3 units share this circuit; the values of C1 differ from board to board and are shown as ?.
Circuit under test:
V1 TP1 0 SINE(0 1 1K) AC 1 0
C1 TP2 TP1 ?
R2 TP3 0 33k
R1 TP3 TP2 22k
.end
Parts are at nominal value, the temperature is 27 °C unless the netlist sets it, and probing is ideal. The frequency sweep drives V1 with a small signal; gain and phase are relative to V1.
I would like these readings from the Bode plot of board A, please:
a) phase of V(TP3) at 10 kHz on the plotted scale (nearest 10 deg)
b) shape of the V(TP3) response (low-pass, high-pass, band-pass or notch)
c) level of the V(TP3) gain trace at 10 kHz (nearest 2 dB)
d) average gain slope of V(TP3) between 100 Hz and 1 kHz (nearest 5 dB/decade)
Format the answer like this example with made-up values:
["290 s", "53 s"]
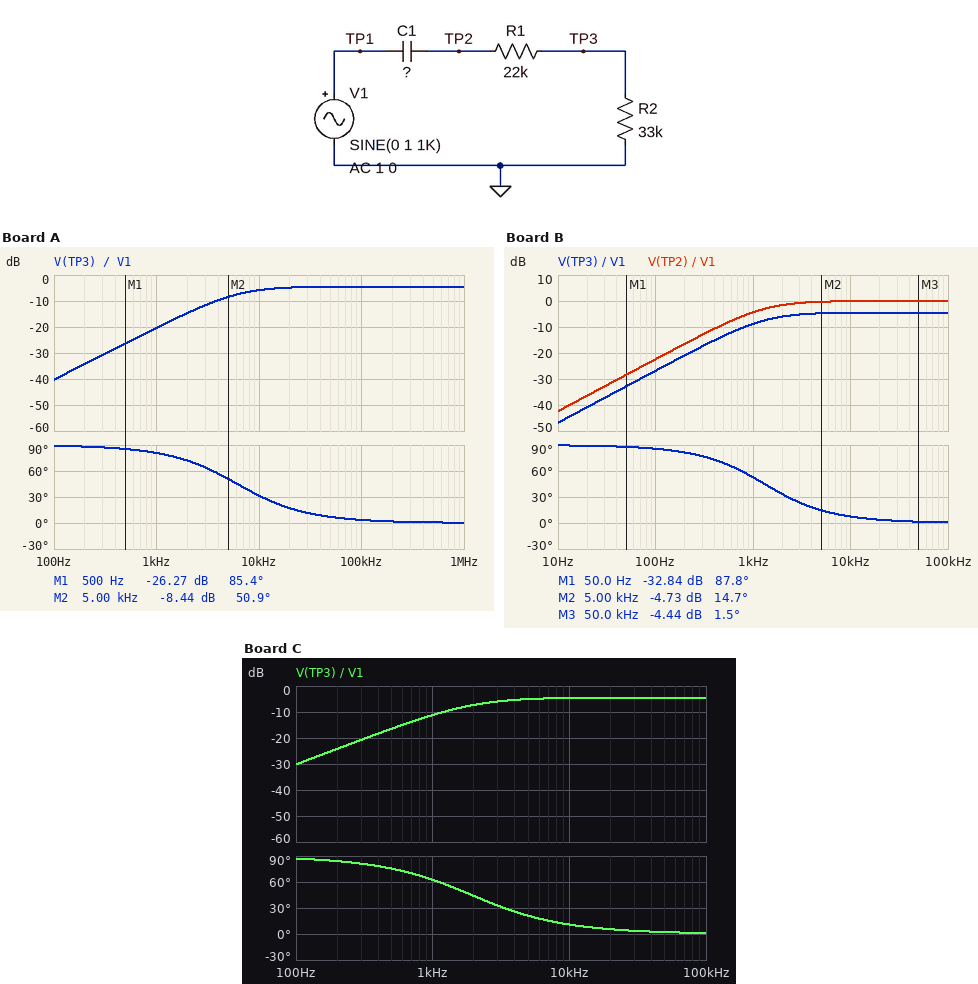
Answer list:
["30 deg", "high-pass", "-6 dB", "20 dB/decade"]
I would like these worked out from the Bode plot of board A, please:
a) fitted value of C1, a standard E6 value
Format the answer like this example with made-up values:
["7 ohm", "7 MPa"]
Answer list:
["470 pF"]
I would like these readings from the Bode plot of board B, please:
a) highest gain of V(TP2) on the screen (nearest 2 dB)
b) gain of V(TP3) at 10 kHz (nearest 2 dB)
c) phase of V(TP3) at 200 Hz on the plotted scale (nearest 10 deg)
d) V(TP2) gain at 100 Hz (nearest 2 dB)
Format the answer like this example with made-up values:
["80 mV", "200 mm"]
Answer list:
["0 dB", "-4 dB", "80 deg", "-22 dB"]
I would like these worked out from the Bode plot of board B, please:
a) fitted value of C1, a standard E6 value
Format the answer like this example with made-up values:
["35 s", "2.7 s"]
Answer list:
["2.2 nF"]
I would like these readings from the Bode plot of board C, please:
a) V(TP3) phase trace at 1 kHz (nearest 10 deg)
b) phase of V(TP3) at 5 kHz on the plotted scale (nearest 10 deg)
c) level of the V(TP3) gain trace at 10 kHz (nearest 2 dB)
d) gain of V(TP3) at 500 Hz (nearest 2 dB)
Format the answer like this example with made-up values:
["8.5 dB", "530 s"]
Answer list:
["60 deg", "20 deg", "-4 dB", "-16 dB"]
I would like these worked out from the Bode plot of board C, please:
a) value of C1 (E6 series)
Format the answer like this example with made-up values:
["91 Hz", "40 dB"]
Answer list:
["1.5 nF"]
